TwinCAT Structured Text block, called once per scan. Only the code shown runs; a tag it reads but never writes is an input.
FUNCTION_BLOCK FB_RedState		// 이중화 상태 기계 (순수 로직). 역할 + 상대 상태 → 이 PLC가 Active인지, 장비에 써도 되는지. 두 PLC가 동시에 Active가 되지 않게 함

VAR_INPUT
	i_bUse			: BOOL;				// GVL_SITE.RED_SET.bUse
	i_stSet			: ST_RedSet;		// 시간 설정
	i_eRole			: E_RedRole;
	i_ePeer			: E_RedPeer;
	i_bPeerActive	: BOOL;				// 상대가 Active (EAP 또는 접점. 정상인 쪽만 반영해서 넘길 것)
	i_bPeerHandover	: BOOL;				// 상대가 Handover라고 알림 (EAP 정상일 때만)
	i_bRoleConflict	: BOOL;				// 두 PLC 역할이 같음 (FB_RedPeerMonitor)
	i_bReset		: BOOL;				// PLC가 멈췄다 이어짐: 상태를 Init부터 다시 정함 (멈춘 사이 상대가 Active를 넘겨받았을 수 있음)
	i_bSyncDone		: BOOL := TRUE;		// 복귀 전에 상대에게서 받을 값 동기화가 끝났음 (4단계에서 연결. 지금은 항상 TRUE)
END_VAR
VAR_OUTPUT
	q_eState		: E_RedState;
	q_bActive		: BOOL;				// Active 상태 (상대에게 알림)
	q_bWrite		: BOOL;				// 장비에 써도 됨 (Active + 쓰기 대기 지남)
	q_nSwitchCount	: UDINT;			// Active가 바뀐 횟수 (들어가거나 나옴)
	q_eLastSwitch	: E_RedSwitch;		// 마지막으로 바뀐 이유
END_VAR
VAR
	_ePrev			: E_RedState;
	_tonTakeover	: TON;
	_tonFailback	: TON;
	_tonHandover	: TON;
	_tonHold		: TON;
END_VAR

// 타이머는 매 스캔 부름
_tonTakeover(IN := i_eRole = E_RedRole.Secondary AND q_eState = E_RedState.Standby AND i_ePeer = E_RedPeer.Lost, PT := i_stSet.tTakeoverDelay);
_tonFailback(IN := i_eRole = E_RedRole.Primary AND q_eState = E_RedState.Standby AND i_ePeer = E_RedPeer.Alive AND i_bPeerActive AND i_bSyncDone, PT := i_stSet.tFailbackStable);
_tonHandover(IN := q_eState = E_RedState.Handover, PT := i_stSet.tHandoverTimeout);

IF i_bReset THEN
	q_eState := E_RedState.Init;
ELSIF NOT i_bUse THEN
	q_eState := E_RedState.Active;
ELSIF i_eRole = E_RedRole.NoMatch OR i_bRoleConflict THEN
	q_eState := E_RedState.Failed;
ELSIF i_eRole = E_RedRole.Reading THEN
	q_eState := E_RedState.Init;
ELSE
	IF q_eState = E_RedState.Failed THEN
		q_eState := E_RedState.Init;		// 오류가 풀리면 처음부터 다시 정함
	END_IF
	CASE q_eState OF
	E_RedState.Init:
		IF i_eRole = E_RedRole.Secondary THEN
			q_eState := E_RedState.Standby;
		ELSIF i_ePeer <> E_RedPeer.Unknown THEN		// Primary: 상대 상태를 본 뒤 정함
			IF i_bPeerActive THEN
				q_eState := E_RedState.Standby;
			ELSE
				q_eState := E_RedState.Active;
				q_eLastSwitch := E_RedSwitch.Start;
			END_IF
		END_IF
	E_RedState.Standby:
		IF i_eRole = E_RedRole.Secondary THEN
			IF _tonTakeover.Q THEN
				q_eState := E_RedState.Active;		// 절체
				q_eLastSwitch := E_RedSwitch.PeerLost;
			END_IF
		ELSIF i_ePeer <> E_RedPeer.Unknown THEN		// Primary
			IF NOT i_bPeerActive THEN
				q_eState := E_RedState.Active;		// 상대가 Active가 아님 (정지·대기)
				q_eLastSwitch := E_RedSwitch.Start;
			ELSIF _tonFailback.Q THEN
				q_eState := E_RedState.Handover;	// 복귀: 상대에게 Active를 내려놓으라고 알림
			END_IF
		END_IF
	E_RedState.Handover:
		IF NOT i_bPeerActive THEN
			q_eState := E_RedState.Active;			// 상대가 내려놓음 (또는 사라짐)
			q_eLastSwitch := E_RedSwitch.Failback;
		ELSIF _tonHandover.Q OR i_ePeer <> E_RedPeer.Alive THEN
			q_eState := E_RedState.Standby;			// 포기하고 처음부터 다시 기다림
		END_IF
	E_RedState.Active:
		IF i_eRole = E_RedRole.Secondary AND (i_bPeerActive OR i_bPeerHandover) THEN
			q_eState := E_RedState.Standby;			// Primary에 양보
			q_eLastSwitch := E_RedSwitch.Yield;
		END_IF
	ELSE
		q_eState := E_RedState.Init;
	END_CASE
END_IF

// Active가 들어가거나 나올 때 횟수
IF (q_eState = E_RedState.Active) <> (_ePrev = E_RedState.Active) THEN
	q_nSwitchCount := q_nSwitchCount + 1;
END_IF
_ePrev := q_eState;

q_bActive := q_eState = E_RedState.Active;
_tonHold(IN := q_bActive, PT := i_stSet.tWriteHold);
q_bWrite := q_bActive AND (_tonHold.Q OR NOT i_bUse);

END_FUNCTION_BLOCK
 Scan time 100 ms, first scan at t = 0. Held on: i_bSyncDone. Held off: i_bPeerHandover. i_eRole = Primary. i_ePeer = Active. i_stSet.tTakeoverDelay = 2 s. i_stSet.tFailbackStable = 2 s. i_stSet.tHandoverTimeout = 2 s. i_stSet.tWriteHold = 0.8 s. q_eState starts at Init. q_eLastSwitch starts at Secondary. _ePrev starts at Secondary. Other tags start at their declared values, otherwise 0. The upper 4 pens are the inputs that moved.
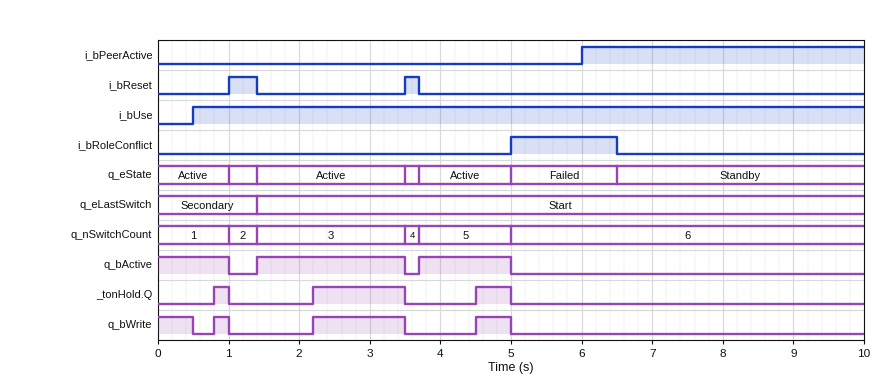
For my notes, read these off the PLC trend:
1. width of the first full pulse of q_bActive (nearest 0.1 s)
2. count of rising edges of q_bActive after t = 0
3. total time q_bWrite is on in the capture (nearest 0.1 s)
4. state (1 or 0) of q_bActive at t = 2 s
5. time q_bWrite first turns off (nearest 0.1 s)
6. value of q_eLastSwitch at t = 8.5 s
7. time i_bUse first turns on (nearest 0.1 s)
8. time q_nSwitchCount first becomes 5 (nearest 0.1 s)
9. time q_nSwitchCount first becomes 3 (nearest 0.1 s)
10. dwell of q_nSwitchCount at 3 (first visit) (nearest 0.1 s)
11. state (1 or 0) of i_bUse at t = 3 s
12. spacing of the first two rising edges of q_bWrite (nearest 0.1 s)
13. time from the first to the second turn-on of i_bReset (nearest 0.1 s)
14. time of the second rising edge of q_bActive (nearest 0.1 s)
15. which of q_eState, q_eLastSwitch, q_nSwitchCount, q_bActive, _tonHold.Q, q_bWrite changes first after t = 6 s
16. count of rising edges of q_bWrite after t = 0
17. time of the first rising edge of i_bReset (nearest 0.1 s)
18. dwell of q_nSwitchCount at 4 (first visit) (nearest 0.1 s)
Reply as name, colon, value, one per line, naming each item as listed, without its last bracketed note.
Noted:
width of the first full pulse of q_bActive: 2.1 s
count of rising edges of q_bActive after t = 0: 2
total time q_bWrite is on in the capture: 2.5 s
state (1 or 0) of q_bActive at t = 2 s: 1
time q_bWrite first turns off: 0.5 s
value of q_eLastSwitch at t = 8.5 s: Start
time i_bUse first turns on: 0.5 s
time q_nSwitchCount first becomes 5: 3.7 s
time q_nSwitchCount first becomes 3: 1.4 s
dwell of q_nSwitchCount at 3 (first visit): 2.1 s
state (1 or 0) of i_bUse at t = 3 s: 1
spacing of the first two rising edges of q_bWrite: 1.4 s
time from the first to the second turn-on of i_bReset: 2.5 s
time of the second rising edge of q_bActive: 3.7 s
which of q_eState, q_eLastSwitch, q_nSwitchCount, q_bActive, _tonHold.Q, q_bWrite changes first after t = 6 s: q_eState
count of rising edges of q_bWrite after t = 0: 3
time of the first rising edge of i_bReset: 1.0 s
dwell of q_nSwitchCount at 4 (first visit): 0.2 s
